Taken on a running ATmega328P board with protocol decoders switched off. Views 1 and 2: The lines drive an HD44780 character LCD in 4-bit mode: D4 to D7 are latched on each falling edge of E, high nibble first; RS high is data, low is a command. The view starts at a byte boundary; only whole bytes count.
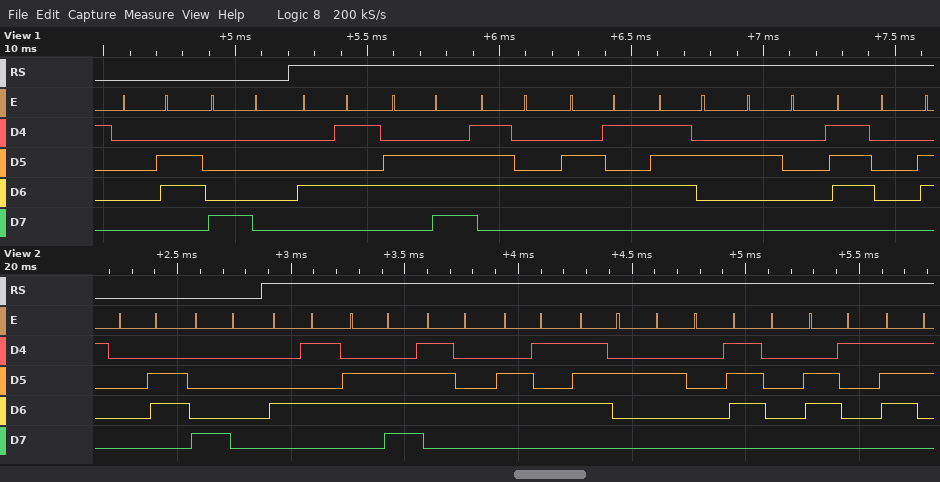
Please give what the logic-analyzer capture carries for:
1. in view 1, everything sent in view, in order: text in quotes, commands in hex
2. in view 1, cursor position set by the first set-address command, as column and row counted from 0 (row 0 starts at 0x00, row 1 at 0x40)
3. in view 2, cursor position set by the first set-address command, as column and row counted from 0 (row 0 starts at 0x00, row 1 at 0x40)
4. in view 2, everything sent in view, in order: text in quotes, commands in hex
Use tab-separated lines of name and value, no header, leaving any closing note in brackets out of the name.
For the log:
in view 1, everything sent in view, in order: text in quotes, commands in hex	0x06 0x80 "Enter p"
in view 1, cursor position set by the first set-address command, as column and row counted from 0	column 0, row 0
in view 2, cursor position set by the first set-address command, as column and row counted from 0	column 0, row 0
in view 2, everything sent in view, in order: text in quotes, commands in hex	0x06 0x80 "Enter pas"
